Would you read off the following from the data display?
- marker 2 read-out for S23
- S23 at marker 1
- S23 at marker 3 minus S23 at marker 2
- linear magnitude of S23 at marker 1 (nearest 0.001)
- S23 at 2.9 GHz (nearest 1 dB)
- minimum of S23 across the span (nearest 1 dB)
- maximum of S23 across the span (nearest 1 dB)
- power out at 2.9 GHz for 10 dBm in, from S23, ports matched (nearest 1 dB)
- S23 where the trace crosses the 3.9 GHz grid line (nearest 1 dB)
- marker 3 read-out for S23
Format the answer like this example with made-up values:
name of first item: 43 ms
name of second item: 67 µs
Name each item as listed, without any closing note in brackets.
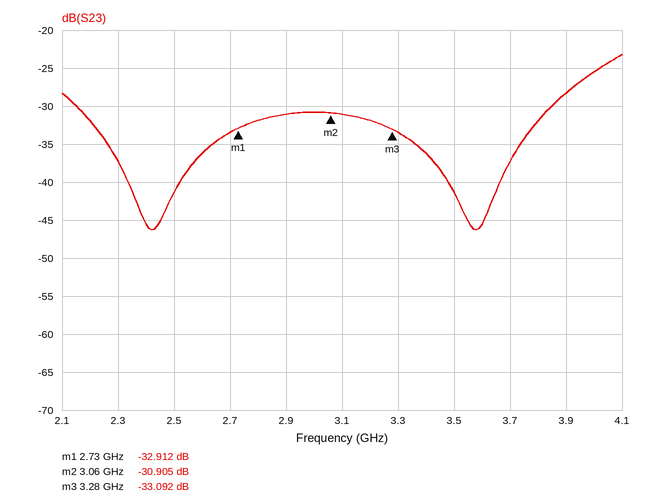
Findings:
marker 2 read-out for S23: -30.905 dB
S23 at marker 1: -32.912 dB
S23 at marker 3 minus S23 at marker 2: -2.187 dB
linear magnitude of S23 at marker 1: 0.023
S23 at 2.9 GHz: -31 dB
minimum of S23 across the span: -46 dB
maximum of S23 across the span: -23 dB
power out at 2.9 GHz for 10 dBm in, from S23, ports matched: -21 dBm
S23 where the trace crosses the 3.9 GHz grid line: -28 dB
marker 3 read-out for S23: -33.092 dB
